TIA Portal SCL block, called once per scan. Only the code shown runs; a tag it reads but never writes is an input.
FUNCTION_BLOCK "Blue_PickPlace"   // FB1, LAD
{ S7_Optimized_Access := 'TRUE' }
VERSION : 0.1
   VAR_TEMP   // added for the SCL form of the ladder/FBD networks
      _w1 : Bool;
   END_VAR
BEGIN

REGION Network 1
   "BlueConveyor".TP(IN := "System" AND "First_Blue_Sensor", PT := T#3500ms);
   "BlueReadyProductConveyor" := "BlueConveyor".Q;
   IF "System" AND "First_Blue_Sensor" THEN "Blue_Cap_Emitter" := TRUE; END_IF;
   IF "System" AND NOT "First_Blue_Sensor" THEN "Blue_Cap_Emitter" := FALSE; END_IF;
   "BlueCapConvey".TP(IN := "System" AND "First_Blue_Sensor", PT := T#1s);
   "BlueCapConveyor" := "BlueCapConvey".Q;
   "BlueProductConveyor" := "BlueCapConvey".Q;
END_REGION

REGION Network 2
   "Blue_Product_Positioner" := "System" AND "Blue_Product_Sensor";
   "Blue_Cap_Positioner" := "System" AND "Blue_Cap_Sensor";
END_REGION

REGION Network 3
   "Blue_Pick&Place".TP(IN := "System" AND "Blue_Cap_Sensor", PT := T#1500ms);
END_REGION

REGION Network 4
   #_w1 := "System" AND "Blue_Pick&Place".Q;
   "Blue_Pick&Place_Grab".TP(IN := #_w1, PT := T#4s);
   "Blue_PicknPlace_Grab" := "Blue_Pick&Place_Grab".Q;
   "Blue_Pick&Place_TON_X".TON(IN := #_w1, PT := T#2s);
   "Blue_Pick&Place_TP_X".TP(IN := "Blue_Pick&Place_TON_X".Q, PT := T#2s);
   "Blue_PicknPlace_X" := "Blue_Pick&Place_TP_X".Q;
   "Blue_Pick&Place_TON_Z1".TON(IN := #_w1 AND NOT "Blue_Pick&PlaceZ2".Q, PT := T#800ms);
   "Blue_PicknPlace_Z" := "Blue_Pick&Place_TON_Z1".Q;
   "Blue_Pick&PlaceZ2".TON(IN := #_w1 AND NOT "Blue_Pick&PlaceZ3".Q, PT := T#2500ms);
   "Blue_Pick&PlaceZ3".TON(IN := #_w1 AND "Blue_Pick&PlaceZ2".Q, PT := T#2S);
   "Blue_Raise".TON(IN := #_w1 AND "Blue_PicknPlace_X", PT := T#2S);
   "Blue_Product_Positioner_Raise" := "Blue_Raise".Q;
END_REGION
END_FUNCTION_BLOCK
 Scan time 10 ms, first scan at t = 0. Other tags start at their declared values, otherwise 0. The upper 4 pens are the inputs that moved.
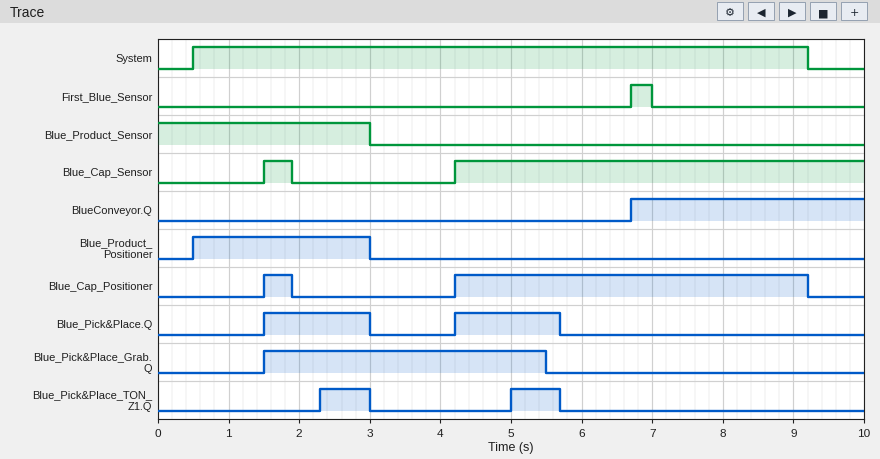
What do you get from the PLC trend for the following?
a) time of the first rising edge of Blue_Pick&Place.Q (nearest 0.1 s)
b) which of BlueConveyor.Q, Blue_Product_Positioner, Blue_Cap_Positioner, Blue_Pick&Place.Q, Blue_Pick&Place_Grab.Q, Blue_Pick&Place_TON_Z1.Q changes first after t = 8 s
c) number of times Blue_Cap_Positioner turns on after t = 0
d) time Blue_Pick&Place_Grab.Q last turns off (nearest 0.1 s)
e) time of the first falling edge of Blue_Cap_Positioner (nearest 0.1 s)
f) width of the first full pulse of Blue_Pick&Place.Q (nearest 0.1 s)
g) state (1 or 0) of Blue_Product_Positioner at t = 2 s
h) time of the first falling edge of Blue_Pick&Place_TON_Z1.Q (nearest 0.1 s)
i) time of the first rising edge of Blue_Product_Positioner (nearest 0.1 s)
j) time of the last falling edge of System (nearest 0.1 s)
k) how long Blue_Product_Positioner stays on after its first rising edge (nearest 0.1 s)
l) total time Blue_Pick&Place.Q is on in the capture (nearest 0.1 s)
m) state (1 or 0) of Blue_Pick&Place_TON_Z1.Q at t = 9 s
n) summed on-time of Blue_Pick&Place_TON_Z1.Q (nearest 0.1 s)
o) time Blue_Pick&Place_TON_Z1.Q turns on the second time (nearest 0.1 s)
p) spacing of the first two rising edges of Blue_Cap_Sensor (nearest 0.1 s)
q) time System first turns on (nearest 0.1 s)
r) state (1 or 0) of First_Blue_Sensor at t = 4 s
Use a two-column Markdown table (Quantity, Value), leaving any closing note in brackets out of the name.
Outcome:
| Quantity | Value |
|---|---|
| time of the first rising edge of Blue_Pick&Place.Q | 1.5 s |
| which of BlueConveyor.Q, Blue_Product_Positioner, Blue_Cap_Positioner, Blue_Pick&Place.Q, Blue_Pick&Place_Grab.Q, Blue_Pick&Place_TON_Z1.Q changes first after t = 8 s | Blue_Cap_Positioner |
| number of times Blue_Cap_Positioner turns on after t = 0 | 2 |
| time Blue_Pick&Place_Grab.Q last turns off | 5.5 s |
| time of the first falling edge of Blue_Cap_Positioner | 1.9 s |
| width of the first full pulse of Blue_Pick&Place.Q | 1.5 s |
| state (1 or 0) of Blue_Product_Positioner at t = 2 s | 1 |
| time of the first falling edge of Blue_Pick&Place_TON_Z1.Q | 3.0 s |
| time of the first rising edge of Blue_Product_Positioner | 0.5 s |
| time of the last falling edge of System | 9.2 s |
| how long Blue_Product_Positioner stays on after its first rising edge | 2.5 s |
| total time Blue_Pick&Place.Q is on in the capture | 3.0 s |
| state (1 or 0) of Blue_Pick&Place_TON_Z1.Q at t = 9 s | 0 |
| summed on-time of Blue_Pick&Place_TON_Z1.Q | 1.4 s |
| time Blue_Pick&Place_TON_Z1.Q turns on the second time | 5.0 s |
| spacing of the first two rising edges of Blue_Cap_Sensor | 2.7 s |
| time System first turns on | 0.5 s |
| state (1 or 0) of First_Blue_Sensor at t = 4 s | 0 |
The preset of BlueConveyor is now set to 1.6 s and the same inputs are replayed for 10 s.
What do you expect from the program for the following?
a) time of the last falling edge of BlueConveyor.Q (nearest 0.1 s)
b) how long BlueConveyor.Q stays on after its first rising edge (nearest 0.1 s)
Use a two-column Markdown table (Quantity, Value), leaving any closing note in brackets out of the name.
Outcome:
| Quantity | Value |
|---|---|
| time of the last falling edge of BlueConveyor.Q | 8.3 s |
| how long BlueConveyor.Q stays on after its first rising edge | 1.6 s |
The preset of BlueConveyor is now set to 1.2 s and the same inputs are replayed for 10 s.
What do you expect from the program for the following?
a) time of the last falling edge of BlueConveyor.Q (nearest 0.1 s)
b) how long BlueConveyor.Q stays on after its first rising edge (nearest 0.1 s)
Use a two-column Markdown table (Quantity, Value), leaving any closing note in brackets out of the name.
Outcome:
| Quantity | Value |
|---|---|
| time of the last falling edge of BlueConveyor.Q | 7.9 s |
| how long BlueConveyor.Q stays on after its first rising edge | 1.2 s |
